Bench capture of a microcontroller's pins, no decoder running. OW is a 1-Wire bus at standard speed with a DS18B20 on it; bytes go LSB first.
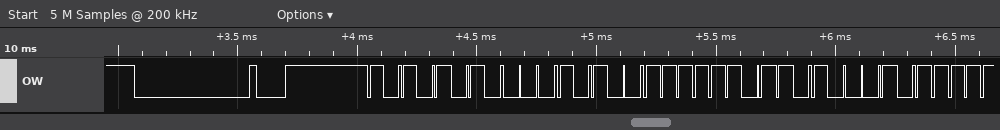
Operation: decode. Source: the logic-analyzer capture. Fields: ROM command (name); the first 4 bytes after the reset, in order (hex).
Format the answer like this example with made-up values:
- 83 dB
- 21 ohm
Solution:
- Match ROM
- 55 28 BF 45
